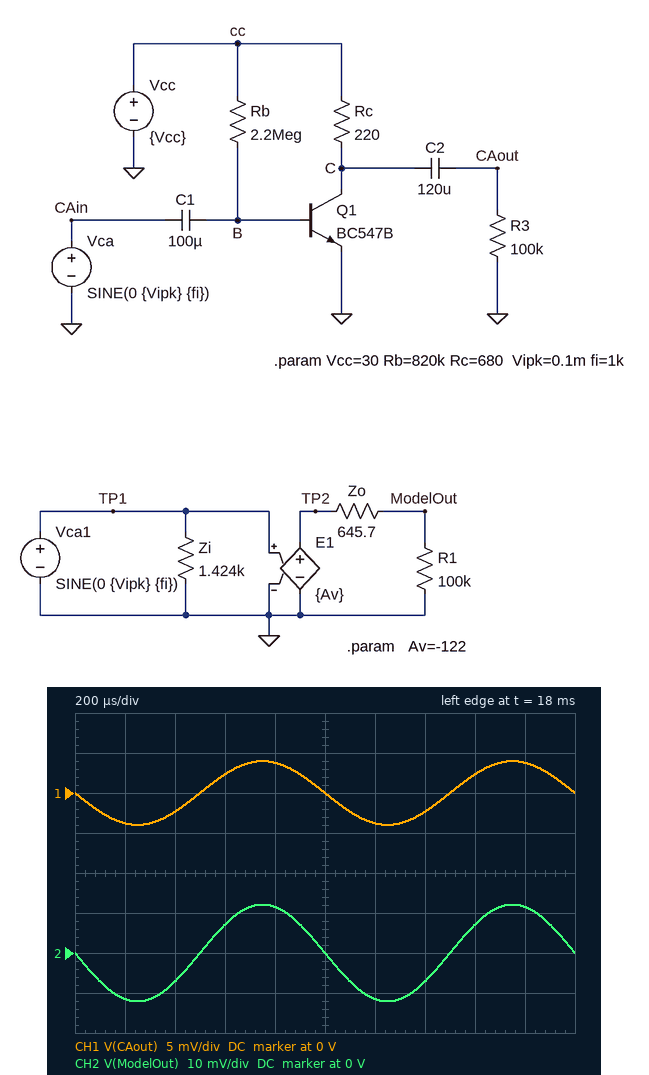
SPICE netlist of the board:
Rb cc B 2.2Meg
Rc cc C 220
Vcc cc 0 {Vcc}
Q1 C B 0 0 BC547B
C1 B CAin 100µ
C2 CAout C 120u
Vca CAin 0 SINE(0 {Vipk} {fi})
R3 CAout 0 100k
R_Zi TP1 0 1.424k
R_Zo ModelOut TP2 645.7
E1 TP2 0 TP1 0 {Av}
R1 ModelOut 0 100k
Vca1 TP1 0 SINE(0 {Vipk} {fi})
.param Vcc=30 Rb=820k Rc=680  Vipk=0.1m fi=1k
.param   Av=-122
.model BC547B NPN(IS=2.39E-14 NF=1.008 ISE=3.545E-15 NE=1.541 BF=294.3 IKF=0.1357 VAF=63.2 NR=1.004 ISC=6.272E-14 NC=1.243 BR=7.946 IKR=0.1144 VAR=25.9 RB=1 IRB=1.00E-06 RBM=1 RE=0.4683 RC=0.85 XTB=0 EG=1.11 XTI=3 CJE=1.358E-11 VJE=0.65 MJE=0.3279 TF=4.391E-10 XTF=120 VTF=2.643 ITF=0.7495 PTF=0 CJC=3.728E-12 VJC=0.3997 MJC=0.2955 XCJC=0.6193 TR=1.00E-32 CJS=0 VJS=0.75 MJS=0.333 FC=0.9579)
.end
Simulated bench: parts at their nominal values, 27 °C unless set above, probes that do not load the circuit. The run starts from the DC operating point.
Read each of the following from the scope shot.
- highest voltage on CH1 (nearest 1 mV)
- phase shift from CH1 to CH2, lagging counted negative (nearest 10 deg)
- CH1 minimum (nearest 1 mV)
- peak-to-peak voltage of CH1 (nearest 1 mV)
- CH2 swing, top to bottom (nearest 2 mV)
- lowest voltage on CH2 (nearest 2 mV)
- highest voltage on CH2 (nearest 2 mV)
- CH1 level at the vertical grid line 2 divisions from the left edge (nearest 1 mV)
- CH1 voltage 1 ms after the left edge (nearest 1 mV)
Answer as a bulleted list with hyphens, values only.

- 4 mV
- 0 deg
- -4 mV
- 8 mV
- 24 mV
- -12 mV
- 12 mV
- -2 mV
- 0 V
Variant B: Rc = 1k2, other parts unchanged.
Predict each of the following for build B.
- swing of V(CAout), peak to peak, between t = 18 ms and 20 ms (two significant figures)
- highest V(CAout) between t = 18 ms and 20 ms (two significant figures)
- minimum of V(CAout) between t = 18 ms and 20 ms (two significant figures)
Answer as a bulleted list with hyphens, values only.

- 39 mV
- 19 mV
- -19 mV
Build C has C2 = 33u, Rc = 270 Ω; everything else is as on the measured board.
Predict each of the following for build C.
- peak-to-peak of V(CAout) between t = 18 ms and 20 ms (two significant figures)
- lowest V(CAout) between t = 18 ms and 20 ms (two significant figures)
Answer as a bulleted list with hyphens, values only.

- 9.7 mV
- -4.9 mV
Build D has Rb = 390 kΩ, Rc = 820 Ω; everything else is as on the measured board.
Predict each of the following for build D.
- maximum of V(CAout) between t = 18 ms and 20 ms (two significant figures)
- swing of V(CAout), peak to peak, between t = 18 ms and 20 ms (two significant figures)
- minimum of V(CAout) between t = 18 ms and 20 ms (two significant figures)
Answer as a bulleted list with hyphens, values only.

- 38 mV
- 76 mV
- -38 mV
